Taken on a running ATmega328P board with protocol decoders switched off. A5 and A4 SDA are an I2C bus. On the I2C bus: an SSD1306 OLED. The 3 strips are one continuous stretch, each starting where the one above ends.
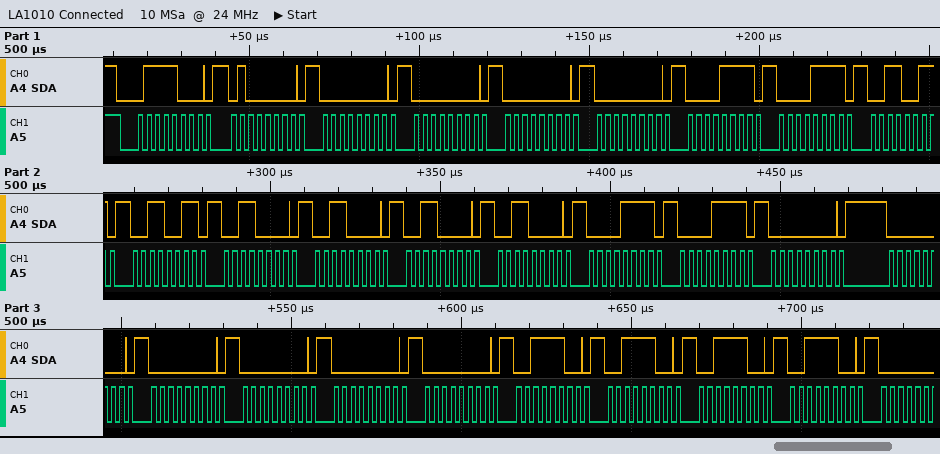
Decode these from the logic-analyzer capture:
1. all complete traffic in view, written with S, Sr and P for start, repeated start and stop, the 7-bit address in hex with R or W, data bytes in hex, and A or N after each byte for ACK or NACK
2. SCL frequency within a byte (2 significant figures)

S 3CW A 40 A 00 A 00 A 00 A 00 A 0F A 0F A 33 A 33 A 30 A 30 A 30 A 30 A 0F A 0F A 00 A 00 A 00 A 00 A 00 A 00 A 3C A 3C A 3C A 3C A
400 kHz
